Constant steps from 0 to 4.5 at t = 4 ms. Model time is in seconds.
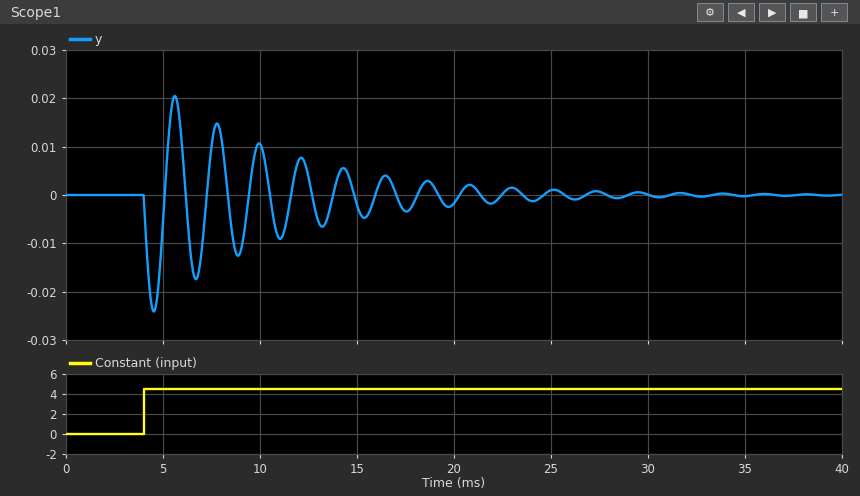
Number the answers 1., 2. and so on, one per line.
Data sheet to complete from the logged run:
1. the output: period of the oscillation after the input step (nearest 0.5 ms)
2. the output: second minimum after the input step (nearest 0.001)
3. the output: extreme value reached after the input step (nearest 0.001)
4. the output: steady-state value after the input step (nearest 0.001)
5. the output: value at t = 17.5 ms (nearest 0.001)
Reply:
1. 2.0 ms
2. -0.017
3. -0.024
4. 0.000
5. -0.003
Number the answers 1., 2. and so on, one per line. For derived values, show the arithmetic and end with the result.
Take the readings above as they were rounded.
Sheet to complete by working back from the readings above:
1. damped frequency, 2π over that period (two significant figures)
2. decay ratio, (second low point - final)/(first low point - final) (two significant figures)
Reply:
1. 2π / 2 = 3.1 rad/ms
2. (-0.017 - 0) / (-0.024 - 0) = 0.71
